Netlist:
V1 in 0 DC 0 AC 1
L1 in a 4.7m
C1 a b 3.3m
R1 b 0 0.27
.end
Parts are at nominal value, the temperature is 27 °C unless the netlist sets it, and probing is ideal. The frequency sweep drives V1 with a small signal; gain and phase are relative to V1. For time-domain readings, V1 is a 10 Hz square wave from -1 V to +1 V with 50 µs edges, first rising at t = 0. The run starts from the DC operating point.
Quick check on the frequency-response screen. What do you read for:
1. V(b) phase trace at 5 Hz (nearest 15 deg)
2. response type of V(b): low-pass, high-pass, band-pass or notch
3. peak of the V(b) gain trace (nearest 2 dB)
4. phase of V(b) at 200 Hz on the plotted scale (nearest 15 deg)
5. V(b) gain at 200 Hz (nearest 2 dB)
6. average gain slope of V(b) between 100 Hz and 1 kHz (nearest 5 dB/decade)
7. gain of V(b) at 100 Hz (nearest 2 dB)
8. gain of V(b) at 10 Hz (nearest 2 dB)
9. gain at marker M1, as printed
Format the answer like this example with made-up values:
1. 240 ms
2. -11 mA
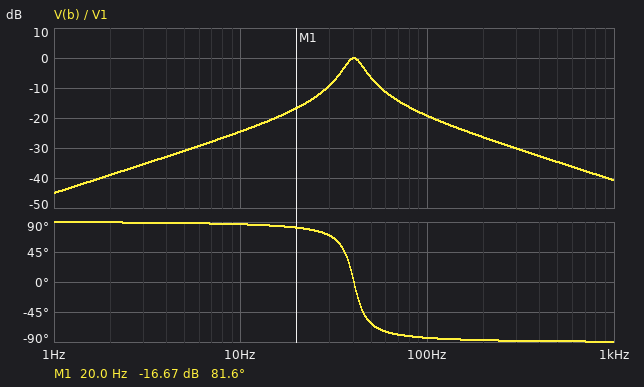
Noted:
1. 90 deg
2. band-pass
3. 0 dB
4. -90 deg
5. -26 dB
6. -20 dB/decade
7. -20 dB
8. -24 dB
9. -16.67 dB
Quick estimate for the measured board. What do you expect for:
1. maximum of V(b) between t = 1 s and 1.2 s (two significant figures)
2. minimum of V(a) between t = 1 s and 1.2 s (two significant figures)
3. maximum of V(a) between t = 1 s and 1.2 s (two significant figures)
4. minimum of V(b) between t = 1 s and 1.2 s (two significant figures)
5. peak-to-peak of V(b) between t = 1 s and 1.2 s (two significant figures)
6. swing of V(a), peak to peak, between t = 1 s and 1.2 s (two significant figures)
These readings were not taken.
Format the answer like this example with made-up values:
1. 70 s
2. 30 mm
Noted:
1. 310 mV
2. -2.2 V
3. 2.2 V
4. -310 mV
5. 620 mV
6. 4.3 V
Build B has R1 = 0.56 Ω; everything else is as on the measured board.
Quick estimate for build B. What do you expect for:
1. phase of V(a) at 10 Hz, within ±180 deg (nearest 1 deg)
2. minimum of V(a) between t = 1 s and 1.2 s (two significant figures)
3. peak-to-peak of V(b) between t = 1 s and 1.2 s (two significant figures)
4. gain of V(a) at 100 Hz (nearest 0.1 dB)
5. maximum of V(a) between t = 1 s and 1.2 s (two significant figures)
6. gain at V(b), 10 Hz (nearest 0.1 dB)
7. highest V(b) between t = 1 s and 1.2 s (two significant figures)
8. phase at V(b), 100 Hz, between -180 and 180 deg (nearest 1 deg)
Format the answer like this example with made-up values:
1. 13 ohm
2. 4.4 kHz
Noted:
1. 0 deg
2. -2.0 V
3. 1.3 V
4. -10.7 dB
5. 2.0 V
6. -18.2 dB
7. 650 mV
8. -77 deg
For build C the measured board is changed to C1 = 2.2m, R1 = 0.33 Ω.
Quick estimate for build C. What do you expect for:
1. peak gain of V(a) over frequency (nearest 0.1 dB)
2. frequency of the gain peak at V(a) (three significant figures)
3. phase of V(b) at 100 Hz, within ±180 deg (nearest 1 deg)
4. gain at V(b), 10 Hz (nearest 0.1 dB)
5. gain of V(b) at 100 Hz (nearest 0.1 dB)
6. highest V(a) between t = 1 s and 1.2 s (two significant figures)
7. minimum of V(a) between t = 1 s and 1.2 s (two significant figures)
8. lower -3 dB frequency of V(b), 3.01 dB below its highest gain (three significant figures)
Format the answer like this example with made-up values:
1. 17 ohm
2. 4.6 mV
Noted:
1. 13.2 dB
2. 48.9 Hz
3. -82 deg
4. -26.5 dB
5. -16.7 dB
6. 2.7 V
7. -2.7 V
8. 44.2 Hz
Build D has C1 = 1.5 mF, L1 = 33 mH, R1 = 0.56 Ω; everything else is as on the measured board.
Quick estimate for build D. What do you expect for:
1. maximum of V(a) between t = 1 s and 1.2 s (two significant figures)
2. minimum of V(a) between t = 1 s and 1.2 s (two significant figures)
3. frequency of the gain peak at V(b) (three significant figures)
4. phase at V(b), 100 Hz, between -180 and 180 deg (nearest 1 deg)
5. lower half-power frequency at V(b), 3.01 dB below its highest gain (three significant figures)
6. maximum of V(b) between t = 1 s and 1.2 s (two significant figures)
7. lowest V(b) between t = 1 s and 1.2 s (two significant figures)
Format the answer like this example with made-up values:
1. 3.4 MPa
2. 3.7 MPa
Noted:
1. 2.1 V
2. -2.1 V
3. 22.6 Hz
4. -88 deg
5. 21.3 Hz
6. 140 mV
7. -140 mV
